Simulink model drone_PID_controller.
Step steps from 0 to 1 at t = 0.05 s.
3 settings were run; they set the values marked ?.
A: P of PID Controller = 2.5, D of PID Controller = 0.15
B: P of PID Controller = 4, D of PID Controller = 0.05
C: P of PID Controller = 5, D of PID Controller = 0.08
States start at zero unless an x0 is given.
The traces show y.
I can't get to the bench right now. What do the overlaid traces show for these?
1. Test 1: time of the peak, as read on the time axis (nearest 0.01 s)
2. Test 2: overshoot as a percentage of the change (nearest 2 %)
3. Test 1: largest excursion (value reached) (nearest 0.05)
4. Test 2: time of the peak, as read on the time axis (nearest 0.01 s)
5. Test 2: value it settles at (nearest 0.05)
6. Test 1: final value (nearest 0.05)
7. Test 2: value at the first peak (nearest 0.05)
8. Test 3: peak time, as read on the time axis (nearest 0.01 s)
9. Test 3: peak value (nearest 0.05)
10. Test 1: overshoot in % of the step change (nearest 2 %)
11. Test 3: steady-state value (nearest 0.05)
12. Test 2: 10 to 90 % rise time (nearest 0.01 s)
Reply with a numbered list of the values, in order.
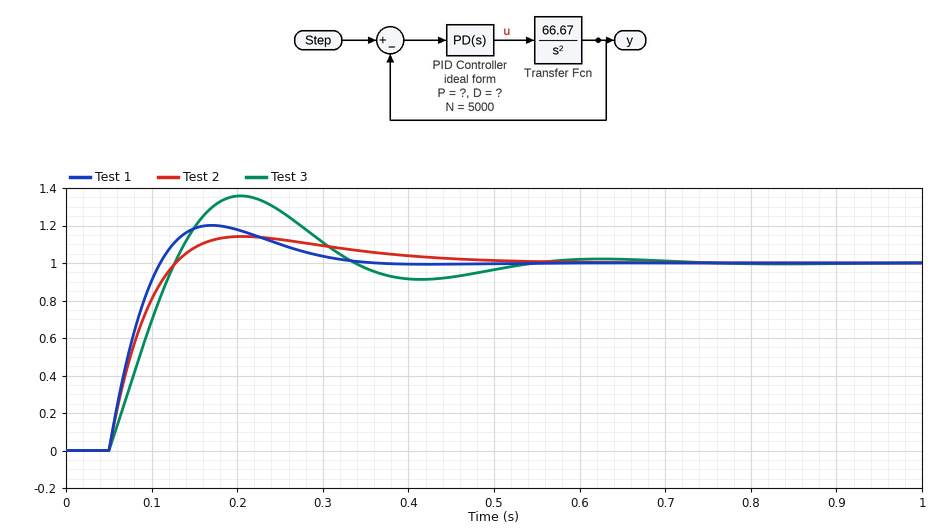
1. 0.17 s
2. 14 %
3. 1.20
4. 0.21 s
5. 1.00
6. 1.00
7. 1.15
8. 0.20 s
9. 1.35
10. 20 %
11. 1.00
12. 0.06 s
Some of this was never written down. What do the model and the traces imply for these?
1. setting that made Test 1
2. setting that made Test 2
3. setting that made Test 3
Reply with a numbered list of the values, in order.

1. C
2. A
3. B
